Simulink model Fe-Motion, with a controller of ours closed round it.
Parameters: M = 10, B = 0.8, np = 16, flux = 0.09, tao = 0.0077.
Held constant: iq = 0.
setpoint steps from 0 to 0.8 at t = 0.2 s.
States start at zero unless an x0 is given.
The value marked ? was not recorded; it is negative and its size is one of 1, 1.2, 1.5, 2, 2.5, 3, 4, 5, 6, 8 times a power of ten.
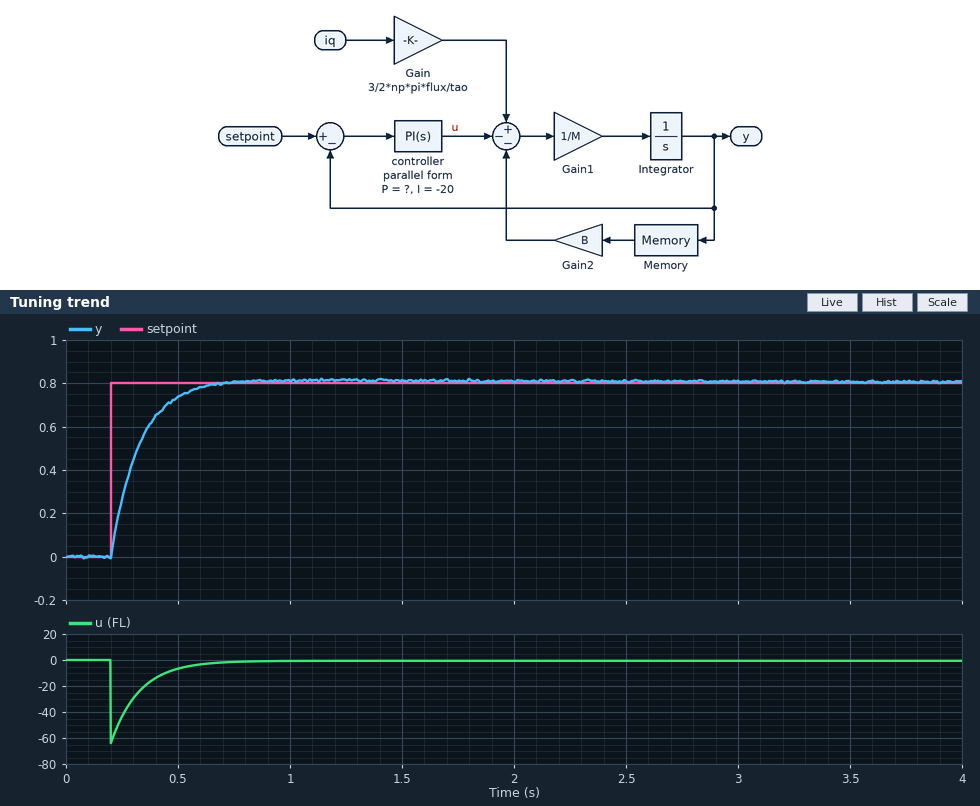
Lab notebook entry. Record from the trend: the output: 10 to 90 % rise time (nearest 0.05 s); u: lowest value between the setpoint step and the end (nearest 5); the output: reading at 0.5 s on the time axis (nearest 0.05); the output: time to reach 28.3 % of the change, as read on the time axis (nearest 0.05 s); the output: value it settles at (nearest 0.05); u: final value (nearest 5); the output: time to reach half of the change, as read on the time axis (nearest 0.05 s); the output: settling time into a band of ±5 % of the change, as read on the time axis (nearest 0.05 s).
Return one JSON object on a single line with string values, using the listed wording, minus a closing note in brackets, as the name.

{"the output: 10 to 90 % rise time": "0.25 s", "u: lowest value between the setpoint step and the end": "-65", "the output: reading at 0.5 s on the time axis": "0.75", "the output: time to reach 28.3 % of the change, as read on the time axis": "0.25 s", "the output: value it settles at": "0.80", "u: final value": "0", "the output: time to reach half of the change, as read on the time axis": "0.30 s", "the output: settling time into a band of ±5 % of the change, as read on the time axis": "0.55 s"}
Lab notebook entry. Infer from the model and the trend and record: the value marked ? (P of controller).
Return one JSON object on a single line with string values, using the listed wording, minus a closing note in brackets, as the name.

{"the value marked ?": "-80"}
